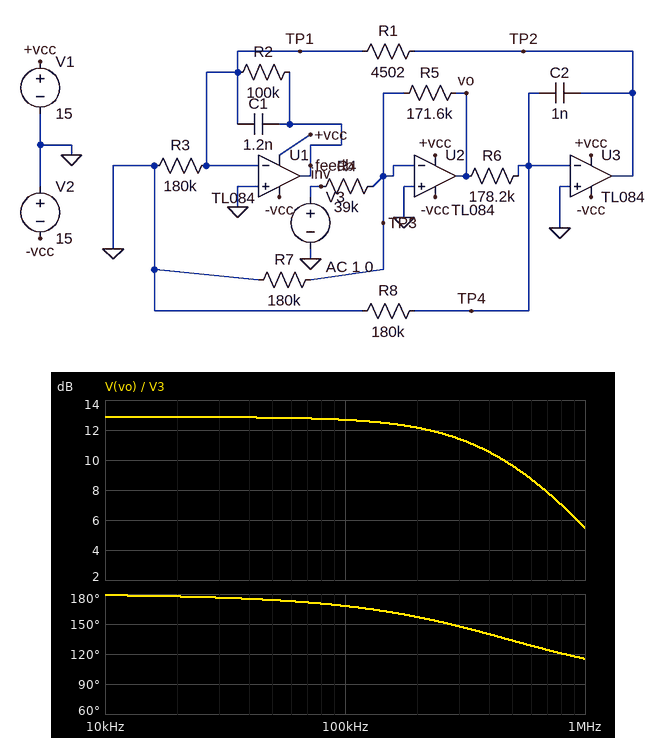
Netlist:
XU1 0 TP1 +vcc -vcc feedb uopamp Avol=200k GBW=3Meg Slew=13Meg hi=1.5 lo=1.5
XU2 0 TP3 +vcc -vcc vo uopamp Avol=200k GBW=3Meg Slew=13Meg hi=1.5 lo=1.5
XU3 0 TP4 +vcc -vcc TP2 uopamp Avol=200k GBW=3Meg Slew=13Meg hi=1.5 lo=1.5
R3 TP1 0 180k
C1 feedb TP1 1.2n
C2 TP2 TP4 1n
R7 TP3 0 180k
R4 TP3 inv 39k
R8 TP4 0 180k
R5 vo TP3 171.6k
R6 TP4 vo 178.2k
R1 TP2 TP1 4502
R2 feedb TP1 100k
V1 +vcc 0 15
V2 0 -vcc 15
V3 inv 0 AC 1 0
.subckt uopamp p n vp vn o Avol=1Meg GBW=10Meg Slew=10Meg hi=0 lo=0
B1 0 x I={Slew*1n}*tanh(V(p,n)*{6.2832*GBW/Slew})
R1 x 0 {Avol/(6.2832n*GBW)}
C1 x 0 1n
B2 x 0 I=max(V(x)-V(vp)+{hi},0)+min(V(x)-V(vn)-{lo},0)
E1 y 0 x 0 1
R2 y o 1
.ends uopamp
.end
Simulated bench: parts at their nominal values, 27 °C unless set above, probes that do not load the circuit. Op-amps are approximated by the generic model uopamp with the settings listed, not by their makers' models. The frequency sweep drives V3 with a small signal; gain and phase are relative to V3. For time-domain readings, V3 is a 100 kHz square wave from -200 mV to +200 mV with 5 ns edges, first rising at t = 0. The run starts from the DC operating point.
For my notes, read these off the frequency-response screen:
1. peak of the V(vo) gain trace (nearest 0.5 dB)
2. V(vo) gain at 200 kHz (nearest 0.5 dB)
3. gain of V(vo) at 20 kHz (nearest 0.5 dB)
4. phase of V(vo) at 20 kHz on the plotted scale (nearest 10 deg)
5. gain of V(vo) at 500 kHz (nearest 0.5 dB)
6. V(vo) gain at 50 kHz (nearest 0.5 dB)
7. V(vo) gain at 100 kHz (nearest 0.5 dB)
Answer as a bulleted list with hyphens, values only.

- 13.0 dB
- 12.0 dB
- 13.0 dB
- 180 deg
- 9.5 dB
- 13.0 dB
- 12.5 dB
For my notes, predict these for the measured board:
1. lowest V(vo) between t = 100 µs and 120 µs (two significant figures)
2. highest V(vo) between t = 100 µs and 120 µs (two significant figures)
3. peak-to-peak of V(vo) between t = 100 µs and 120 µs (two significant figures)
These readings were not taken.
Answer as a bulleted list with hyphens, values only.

- -880 mV
- 880 mV
- 1.8 V
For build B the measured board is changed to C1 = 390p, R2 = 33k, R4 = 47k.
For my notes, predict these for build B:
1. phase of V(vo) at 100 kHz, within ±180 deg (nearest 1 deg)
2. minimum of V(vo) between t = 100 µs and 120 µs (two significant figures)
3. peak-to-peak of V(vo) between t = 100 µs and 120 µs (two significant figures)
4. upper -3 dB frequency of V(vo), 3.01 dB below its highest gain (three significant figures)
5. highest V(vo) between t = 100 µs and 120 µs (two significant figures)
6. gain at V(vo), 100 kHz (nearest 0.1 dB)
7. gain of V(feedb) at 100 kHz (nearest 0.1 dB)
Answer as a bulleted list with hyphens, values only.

- 169 deg
- -730 mV
- 1.5 V
- 535 kHz
- 730 mV
- 11.1 dB
- -31.1 dB
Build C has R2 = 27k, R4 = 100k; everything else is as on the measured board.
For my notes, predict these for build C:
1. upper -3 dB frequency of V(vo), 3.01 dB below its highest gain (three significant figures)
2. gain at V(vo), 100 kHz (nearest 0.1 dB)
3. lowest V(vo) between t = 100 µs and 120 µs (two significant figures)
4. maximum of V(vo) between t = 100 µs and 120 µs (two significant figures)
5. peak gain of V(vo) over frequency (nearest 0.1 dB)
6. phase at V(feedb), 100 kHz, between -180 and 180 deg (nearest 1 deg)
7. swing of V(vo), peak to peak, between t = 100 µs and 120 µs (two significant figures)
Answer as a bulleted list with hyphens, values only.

- 818 kHz
- 4.6 dB
- -340 mV
- 340 mV
- 4.7 dB
- -8 deg
- 690 mV
